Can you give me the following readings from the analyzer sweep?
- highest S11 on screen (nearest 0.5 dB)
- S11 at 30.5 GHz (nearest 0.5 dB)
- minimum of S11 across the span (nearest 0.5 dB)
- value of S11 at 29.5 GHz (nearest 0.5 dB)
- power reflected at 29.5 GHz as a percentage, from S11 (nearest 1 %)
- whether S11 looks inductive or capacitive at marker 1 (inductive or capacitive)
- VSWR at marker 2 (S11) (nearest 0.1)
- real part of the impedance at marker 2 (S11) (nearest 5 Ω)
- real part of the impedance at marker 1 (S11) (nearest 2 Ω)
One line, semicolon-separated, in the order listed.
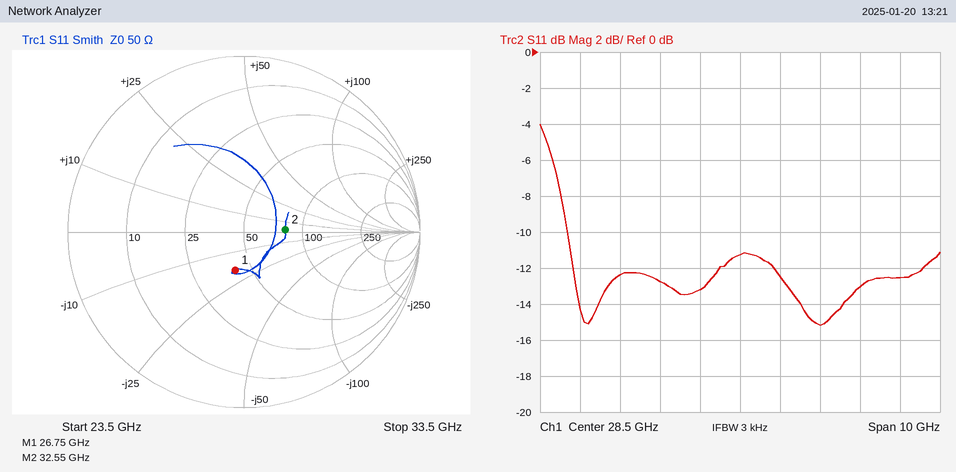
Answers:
-4.0 dB; -15.0 dB; -15.0 dB; -12.5 dB; 6 %; capacitive; 1.6; 80 Ω; 42 Ω
